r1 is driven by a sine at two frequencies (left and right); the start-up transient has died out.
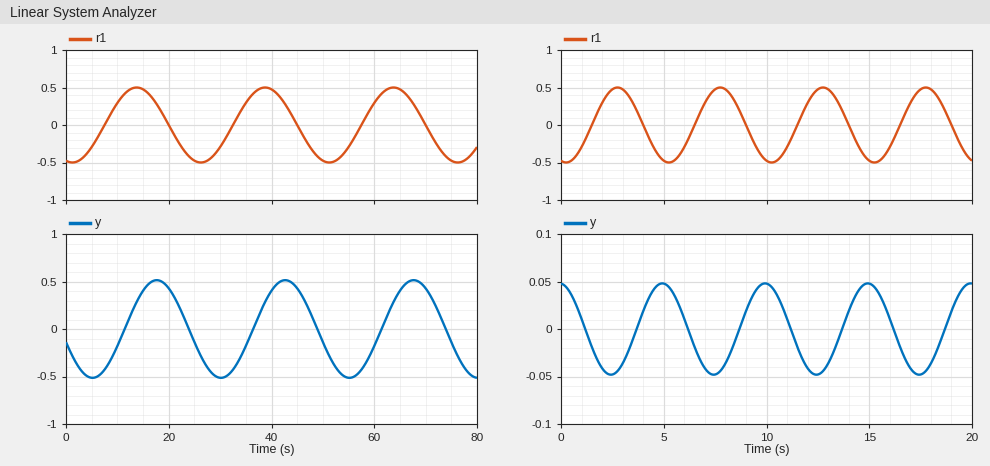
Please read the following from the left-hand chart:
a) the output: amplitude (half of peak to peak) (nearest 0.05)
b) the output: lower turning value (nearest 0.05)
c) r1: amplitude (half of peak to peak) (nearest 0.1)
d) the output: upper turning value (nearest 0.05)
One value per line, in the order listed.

0.50
-0.50
0.5
0.50
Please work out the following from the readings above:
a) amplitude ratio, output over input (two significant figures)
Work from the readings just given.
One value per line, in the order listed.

1.0
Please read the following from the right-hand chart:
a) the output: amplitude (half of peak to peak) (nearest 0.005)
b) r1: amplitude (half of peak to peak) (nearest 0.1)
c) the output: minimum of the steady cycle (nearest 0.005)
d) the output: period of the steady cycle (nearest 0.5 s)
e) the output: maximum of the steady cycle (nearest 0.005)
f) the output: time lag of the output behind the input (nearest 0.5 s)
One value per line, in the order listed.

0.050
0.5
-0.050
5.0 s
0.050
2.0 s
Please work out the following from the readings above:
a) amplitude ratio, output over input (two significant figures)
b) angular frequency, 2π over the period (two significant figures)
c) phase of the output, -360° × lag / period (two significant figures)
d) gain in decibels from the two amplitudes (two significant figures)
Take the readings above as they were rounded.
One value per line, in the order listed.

0.10
1.3 rad/s
-140°
-20 dB
